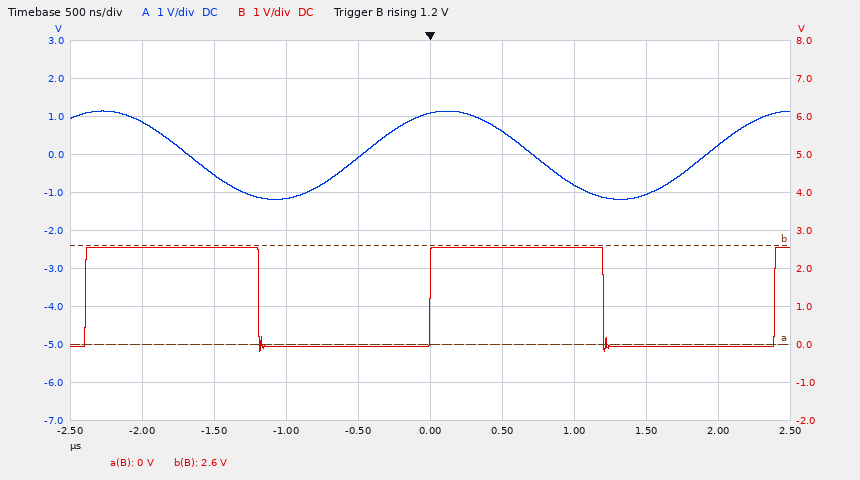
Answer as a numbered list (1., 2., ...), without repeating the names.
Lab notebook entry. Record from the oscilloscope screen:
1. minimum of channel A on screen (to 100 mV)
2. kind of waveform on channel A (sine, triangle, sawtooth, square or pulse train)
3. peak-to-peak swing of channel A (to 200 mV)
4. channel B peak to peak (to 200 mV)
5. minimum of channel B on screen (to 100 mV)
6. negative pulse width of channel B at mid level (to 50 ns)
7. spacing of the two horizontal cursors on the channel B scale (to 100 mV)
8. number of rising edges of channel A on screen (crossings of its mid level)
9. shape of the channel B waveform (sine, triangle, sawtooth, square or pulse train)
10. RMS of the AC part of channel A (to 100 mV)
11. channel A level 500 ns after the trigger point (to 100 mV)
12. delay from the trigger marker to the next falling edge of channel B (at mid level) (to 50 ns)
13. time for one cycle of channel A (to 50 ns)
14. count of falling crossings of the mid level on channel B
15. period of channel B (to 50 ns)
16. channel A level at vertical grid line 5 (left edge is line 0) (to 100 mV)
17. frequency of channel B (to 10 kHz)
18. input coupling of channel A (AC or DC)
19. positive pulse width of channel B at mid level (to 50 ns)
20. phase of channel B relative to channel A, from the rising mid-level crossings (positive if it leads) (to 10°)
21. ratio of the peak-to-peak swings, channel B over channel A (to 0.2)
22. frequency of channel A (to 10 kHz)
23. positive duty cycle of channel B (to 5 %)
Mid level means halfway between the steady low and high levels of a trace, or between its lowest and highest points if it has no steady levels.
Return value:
1. -1.2 V
2. sine
3. 2.4 V
4. 2.8 V
5. -200 mV
6. 1.20 µs
7. 2.6 V
8. 2
9. square
10. 800 mV
11. 600 mV
12. 1.20 µs
13. 2.40 µs
14. 2
15. 2.40 µs
16. 1.1 V
17. 420 kHz
18. DC
19. 1.20 µs
20. -70°
21. 1.2
22. 420 kHz
23. 50 %
